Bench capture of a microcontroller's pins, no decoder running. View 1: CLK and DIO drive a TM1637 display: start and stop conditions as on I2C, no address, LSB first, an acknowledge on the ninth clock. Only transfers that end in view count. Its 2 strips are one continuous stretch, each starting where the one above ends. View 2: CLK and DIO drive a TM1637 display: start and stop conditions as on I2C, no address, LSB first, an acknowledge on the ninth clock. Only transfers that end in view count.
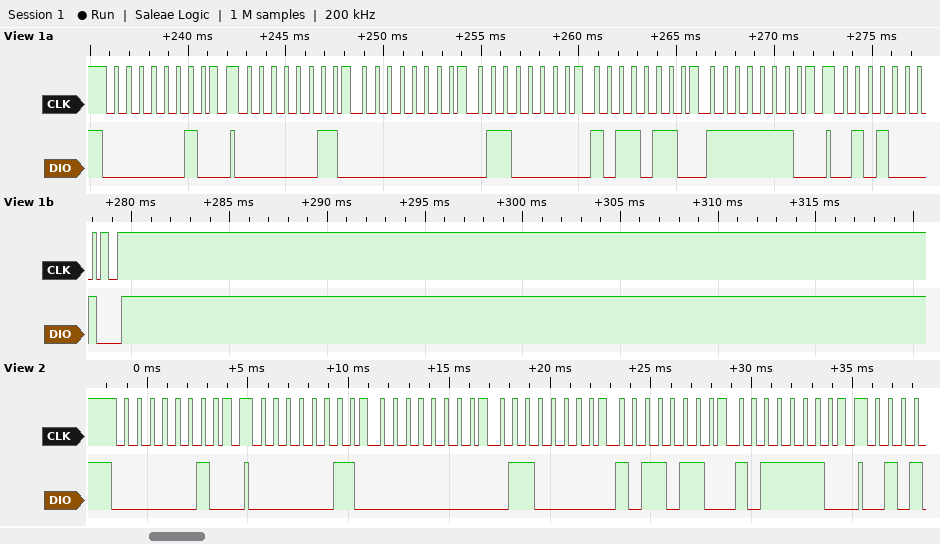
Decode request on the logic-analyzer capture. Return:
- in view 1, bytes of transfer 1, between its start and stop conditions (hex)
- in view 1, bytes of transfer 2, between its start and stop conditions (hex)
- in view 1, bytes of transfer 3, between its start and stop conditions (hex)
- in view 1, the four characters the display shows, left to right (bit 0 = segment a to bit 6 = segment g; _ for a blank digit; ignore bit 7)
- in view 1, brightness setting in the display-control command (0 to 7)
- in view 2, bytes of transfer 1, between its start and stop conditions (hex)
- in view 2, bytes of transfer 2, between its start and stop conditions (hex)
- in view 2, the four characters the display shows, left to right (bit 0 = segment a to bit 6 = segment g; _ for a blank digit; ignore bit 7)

40
C0 00 06 6D 7F
8A
_158
2
40
C0 00 06 6D 7D
_156
